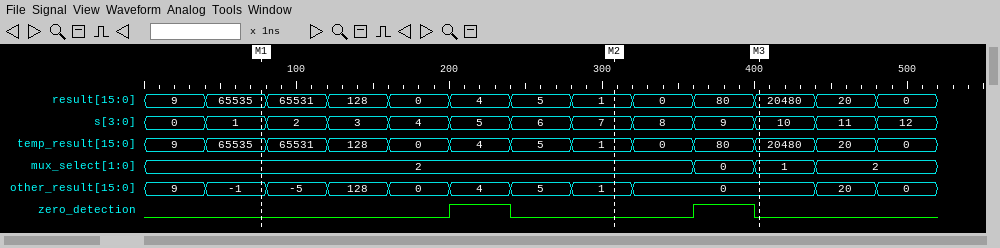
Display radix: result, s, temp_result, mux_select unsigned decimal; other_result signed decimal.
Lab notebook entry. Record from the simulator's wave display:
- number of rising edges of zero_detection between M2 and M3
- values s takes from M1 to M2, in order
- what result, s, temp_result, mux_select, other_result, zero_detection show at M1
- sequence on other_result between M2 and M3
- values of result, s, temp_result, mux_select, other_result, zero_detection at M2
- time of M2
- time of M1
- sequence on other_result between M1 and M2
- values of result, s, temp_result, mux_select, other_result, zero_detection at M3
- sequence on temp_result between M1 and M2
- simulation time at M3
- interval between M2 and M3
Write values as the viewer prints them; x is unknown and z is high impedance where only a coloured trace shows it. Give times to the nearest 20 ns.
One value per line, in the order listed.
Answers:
1
1, 2, 3, 4, 5, 6, 7
result=65535, s=1, temp_result=65535, mux_select=2, other_result=-1, zero_detection=0
1, 0
result=1, s=7, temp_result=1, mux_select=2, other_result=1, zero_detection=0
300 ns
80 ns
-1, -5, 128, 0, 4, 5, 1
result=20480, s=10, temp_result=20480, mux_select=1, other_result=0, zero_detection=0
65535, 65531, 128, 0, 4, 5, 1
400 ns
100 ns
